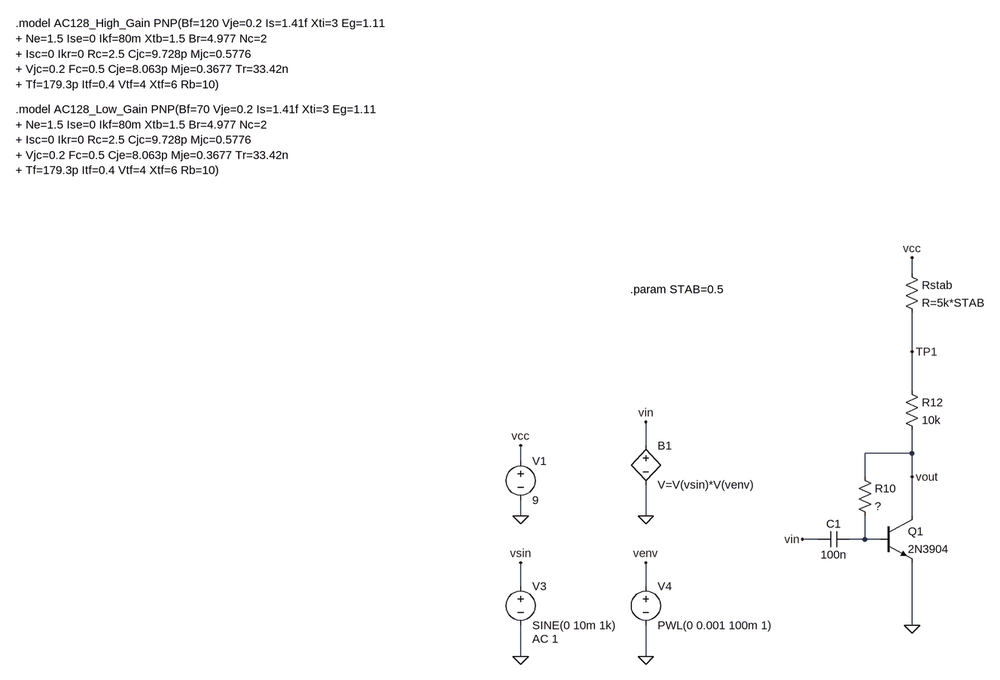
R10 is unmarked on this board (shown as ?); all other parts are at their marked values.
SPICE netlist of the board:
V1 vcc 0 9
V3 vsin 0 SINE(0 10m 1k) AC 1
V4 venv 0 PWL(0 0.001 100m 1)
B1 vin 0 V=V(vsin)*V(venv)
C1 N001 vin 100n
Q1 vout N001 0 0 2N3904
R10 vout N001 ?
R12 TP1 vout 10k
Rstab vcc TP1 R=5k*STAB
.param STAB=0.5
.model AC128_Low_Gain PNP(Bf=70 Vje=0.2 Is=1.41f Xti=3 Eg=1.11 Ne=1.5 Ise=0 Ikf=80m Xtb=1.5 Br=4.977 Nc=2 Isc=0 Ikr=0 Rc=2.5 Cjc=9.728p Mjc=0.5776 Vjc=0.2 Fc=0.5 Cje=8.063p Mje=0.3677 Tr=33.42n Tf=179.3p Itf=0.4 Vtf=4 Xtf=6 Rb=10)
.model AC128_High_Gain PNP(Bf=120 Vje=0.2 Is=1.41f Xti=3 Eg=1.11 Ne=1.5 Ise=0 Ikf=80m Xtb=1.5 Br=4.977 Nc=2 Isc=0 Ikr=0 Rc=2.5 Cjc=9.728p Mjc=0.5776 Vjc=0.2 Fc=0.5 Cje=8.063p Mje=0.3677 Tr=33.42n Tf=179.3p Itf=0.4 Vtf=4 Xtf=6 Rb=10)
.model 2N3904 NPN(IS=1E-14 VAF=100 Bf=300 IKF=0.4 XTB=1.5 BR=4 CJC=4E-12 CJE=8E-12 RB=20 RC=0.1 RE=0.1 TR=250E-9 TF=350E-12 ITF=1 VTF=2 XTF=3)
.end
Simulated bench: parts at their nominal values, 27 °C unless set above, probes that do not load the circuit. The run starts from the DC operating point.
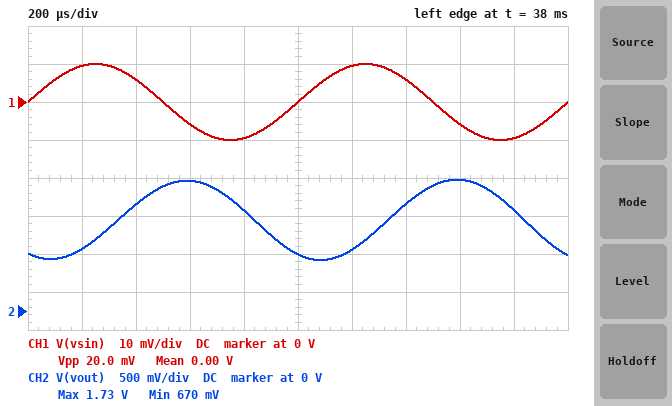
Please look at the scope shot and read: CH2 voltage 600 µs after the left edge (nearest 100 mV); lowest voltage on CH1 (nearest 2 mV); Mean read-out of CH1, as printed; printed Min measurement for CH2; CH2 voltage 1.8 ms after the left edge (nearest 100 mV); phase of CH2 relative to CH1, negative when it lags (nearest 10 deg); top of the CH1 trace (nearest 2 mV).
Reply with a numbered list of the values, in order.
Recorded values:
1. 1.7 V
2. -10 mV
3. 0.00 V
4. 670 mV
5. 1.3 V
6. -120 deg
7. 10 mV
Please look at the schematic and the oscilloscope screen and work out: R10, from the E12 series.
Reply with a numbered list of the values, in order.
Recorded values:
1. 270 kΩ
